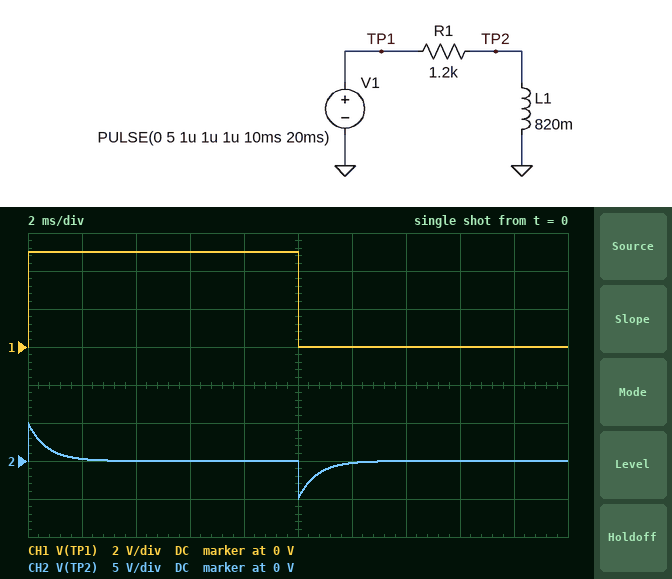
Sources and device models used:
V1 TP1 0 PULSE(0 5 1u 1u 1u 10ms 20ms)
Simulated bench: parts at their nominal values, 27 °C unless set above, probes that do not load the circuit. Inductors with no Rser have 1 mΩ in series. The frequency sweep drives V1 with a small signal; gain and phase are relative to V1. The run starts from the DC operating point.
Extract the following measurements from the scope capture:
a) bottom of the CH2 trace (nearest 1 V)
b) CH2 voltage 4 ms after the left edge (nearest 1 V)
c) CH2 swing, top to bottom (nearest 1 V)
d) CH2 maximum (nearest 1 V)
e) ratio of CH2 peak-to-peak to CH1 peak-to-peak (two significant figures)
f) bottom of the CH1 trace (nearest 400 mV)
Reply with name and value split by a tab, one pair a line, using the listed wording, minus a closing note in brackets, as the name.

bottom of the CH2 trace	-5 V
CH2 voltage 4 ms after the left edge	0 V
CH2 swing, top to bottom	10 V
CH2 maximum	5 V
ratio of CH2 peak-to-peak to CH1 peak-to-peak	2.0
bottom of the CH1 trace	0 V
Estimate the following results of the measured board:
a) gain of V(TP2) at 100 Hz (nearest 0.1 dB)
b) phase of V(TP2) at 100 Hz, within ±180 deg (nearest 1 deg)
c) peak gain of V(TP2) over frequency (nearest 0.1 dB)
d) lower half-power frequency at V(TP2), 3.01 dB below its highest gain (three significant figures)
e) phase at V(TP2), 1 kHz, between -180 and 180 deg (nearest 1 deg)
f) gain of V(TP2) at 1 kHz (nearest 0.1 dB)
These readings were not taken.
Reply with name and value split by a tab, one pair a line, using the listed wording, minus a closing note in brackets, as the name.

gain of V(TP2) at 100 Hz	-8.1 dB
phase of V(TP2) at 100 Hz, within ±180 deg	67 deg
peak gain of V(TP2) over frequency	0 dB
lower half-power frequency at V(TP2), 3.01 dB below its highest gain	233 Hz
phase at V(TP2), 1 kHz, between -180 and 180 deg	13 deg
gain of V(TP2) at 1 kHz	-0.2 dB
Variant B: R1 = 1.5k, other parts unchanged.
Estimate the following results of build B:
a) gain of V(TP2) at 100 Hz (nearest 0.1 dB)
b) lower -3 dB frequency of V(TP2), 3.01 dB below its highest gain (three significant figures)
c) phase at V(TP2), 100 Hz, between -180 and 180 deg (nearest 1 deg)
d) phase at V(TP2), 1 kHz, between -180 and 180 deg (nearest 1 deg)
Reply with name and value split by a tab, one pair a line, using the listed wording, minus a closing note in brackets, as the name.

gain of V(TP2) at 100 Hz	-9.8 dB
lower -3 dB frequency of V(TP2), 3.01 dB below its highest gain	291 Hz
phase at V(TP2), 100 Hz, between -180 and 180 deg	71 deg
phase at V(TP2), 1 kHz, between -180 and 180 deg	16 deg
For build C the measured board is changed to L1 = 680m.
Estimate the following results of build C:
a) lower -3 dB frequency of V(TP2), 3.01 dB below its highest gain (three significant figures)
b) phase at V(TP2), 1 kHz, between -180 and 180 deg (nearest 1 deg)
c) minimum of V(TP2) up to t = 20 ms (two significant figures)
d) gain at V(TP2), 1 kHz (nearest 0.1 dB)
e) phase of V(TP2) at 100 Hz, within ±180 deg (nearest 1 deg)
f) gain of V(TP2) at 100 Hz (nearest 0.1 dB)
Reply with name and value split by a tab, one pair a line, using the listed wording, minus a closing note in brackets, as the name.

lower -3 dB frequency of V(TP2), 3.01 dB below its highest gain	281 Hz
phase at V(TP2), 1 kHz, between -180 and 180 deg	16 deg
minimum of V(TP2) up to t = 20 ms	-5.0 V
gain at V(TP2), 1 kHz	-0.3 dB
phase of V(TP2) at 100 Hz, within ±180 deg	70 deg
gain of V(TP2) at 100 Hz	-9.5 dB
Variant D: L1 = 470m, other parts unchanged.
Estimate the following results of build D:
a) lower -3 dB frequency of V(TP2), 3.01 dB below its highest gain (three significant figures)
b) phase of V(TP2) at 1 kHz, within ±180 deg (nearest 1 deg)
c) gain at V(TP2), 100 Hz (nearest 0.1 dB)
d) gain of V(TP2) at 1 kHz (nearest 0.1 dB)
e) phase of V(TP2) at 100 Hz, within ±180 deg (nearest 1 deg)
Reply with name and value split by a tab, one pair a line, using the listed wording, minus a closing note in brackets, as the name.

lower -3 dB frequency of V(TP2), 3.01 dB below its highest gain	406 Hz
phase of V(TP2) at 1 kHz, within ±180 deg	22 deg
gain at V(TP2), 100 Hz	-12.4 dB
gain of V(TP2) at 1 kHz	-0.7 dB
phase of V(TP2) at 100 Hz, within ±180 deg	76 deg
